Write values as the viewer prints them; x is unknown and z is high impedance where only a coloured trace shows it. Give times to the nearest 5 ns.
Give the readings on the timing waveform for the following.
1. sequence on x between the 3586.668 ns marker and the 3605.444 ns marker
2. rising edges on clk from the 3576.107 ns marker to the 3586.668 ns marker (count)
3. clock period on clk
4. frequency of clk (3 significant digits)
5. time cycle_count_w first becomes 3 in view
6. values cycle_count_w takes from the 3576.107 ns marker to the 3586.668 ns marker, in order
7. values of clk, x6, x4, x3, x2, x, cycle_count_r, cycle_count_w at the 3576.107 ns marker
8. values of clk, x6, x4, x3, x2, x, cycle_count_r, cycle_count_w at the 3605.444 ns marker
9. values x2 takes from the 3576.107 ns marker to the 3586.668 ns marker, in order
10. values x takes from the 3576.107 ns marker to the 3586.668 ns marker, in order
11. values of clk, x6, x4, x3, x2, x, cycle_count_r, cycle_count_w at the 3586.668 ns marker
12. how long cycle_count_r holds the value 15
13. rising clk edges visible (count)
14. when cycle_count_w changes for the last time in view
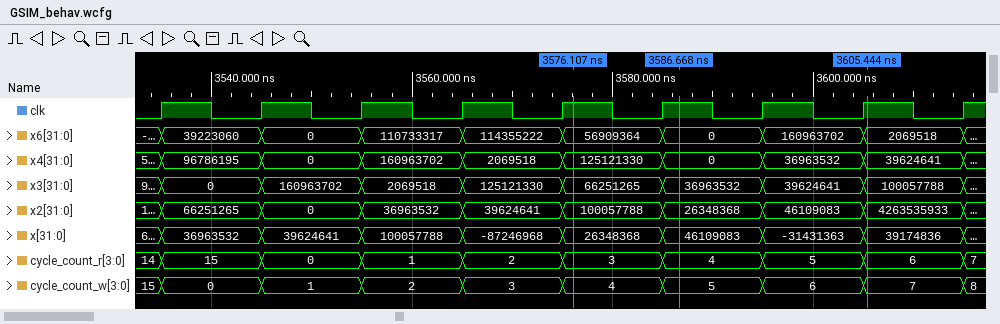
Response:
46109083, -31431363, 39174836
1
10 ns
100 MHz
3565 ns
4, 5
clk=1, x6=56909364, x4=125121330, x3=66251265, x2=100057788, x=26348368, cycle_count_r=3, cycle_count_w=4
clk=1, x6=2069518, x4=39624641, x3=100057788, x2=4263535933, x=39174836, cycle_count_r=6, cycle_count_w=7
100057788, 26348368
26348368, 46109083
clk=1, x6=0, x4=0, x3=36963532, x2=26348368, x=46109083, cycle_count_r=4, cycle_count_w=5
10 ns
9
3615 ns
